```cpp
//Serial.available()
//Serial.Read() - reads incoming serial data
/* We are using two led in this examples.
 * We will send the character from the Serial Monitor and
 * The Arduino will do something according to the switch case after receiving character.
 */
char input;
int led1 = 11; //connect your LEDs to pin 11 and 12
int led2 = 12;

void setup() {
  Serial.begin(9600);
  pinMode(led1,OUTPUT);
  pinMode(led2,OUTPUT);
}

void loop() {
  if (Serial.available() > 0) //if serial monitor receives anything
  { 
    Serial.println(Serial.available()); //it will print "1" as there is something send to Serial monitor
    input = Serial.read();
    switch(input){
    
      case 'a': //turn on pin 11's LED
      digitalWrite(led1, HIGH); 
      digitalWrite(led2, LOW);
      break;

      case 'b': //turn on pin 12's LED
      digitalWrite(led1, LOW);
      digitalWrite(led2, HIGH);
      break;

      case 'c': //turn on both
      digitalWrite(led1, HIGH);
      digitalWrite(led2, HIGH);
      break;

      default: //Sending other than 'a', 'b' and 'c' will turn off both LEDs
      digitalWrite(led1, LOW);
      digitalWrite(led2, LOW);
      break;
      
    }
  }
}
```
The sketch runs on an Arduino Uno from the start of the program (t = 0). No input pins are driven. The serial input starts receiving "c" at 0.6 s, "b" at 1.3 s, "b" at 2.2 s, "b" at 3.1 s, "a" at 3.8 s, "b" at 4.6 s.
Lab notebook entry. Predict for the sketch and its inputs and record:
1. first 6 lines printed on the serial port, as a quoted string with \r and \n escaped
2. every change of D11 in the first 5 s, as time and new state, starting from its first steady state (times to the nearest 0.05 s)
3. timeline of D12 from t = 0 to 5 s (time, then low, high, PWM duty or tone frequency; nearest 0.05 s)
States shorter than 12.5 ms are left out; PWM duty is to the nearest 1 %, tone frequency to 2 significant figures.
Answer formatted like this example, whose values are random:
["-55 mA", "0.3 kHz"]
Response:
["\"1\\r\\n1\\r\\n1\\r\\n1\\r\\n1\\r\\n1\\r\\n\"", "0 s low; 0.6 s high; 1.3 s low; 3.8 s high; 4.6 s low", "0 s low; 0.6 s high; 3.8 s low; 4.6 s high"]
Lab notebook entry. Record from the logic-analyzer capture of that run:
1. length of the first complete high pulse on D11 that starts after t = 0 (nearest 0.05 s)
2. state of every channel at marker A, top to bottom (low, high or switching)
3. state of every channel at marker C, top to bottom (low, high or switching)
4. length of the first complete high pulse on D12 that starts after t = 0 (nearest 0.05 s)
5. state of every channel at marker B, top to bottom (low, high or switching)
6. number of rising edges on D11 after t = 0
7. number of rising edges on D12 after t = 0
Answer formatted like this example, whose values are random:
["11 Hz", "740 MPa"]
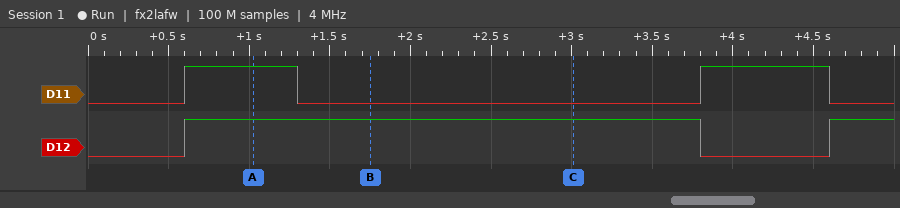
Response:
["0.70 s", "D11 high, D12 high", "D11 low, D12 high", "3.20 s", "D11 low, D12 high", "2", "2"]
